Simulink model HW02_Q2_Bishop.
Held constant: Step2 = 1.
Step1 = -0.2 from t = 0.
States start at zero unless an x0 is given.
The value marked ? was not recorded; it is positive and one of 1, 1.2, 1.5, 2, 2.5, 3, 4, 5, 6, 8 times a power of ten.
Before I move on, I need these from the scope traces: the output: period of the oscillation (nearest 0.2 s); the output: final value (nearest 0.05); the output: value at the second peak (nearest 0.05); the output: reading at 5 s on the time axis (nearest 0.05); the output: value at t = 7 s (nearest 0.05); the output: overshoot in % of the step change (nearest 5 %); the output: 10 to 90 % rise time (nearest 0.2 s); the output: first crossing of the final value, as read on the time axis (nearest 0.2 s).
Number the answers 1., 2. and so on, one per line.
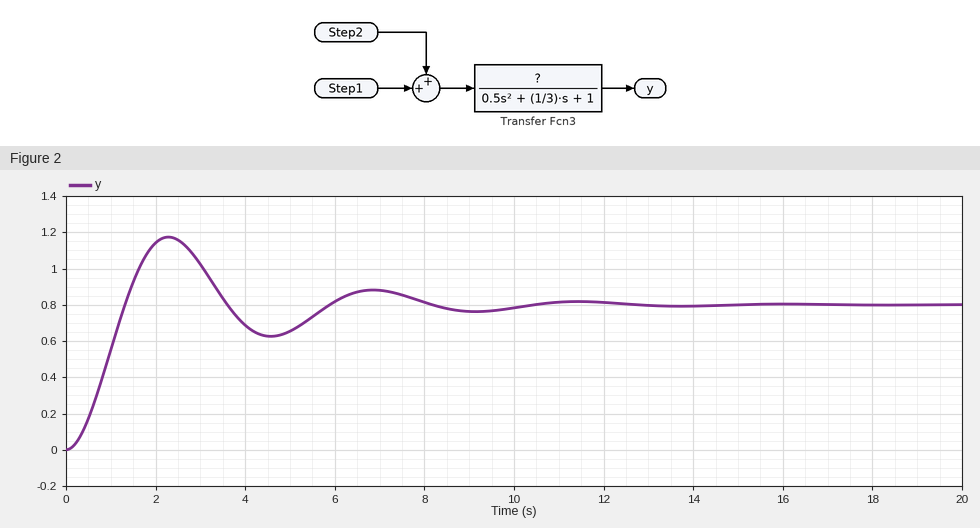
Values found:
1. 4.6 s
2. 0.80
3. 0.90
4. 0.65
5. 0.90
6. 45 %
7. 0.8 s
8. 1.4 s
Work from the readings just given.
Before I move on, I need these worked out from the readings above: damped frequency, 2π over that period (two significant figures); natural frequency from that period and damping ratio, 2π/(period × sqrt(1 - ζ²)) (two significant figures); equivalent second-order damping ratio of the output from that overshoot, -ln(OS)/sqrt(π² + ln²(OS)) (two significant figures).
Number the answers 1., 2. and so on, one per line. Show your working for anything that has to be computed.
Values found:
1. 2π / 4.6 = 1.4 rad/s
2. 2π / (4.6 × sqrt(1 - 0.25²)) = 1.4 rad/s
3. ln(0.45) = -0.799; 0.799 / sqrt(9.870 + 0.638) = 0.25
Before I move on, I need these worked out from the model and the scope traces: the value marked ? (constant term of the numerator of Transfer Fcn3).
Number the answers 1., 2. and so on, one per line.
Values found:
1. 1
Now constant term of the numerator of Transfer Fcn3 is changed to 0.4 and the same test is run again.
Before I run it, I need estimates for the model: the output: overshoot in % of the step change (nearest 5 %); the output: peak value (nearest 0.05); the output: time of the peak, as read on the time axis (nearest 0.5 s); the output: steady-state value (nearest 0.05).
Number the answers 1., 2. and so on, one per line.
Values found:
1. 45 %
2. 0.45
3. 2.5 s
4. 0.30
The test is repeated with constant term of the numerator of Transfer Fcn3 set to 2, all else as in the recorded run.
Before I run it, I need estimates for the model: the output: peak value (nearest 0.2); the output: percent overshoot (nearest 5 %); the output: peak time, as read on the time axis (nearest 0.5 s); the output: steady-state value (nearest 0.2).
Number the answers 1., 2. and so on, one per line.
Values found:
1. 2.4
2. 45 %
3. 2.5 s
4. 1.6
